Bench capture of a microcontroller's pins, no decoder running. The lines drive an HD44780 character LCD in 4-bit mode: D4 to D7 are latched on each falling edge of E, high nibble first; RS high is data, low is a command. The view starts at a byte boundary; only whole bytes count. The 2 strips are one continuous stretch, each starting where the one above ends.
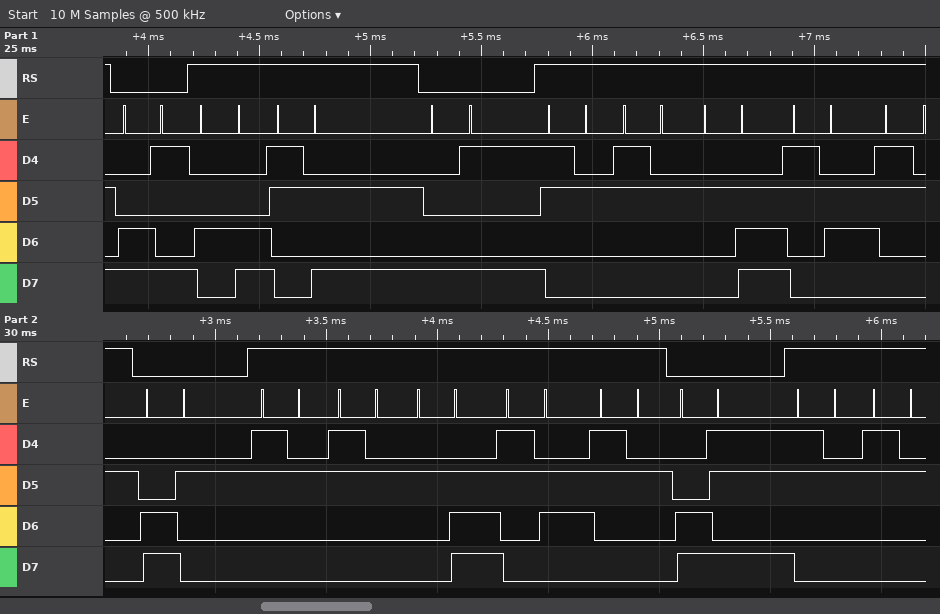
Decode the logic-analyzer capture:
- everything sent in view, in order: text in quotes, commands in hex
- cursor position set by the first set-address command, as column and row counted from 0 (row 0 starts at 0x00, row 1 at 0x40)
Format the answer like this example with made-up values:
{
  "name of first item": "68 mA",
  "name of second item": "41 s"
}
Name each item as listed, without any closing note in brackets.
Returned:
{
  "everything sent in view, in order: text in quotes, commands in hex": "0xC9 \"L:\" 0x89 \"22.62\" 0xC2 \"22.62\" 0xCB \"22\"",
  "cursor position set by the first set-address command, as column and row counted from 0": "column 9, row 1"
}
